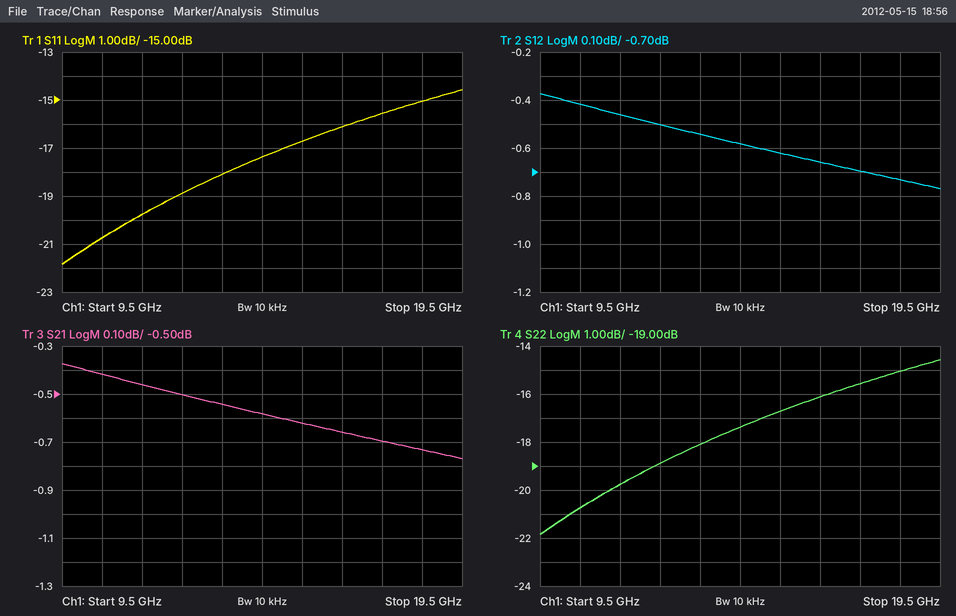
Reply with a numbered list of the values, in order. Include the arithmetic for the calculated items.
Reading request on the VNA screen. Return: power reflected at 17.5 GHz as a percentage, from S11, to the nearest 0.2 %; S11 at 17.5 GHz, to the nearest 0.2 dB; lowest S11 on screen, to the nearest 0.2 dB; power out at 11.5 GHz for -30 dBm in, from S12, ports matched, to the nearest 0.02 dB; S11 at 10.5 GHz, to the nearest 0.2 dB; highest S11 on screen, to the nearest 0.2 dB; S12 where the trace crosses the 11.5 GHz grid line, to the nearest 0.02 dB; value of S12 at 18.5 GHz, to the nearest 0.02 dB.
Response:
1. 10^(-15.6/10) ≈ 2.8 %
2. -15.6 dB
3. -21.8 dB
4. -30 dBm + (-0.46 dB) = -30.46 dBm
5. -20.8 dB
6. -14.6 dB
7. -0.46 dB
8. -0.74 dB
